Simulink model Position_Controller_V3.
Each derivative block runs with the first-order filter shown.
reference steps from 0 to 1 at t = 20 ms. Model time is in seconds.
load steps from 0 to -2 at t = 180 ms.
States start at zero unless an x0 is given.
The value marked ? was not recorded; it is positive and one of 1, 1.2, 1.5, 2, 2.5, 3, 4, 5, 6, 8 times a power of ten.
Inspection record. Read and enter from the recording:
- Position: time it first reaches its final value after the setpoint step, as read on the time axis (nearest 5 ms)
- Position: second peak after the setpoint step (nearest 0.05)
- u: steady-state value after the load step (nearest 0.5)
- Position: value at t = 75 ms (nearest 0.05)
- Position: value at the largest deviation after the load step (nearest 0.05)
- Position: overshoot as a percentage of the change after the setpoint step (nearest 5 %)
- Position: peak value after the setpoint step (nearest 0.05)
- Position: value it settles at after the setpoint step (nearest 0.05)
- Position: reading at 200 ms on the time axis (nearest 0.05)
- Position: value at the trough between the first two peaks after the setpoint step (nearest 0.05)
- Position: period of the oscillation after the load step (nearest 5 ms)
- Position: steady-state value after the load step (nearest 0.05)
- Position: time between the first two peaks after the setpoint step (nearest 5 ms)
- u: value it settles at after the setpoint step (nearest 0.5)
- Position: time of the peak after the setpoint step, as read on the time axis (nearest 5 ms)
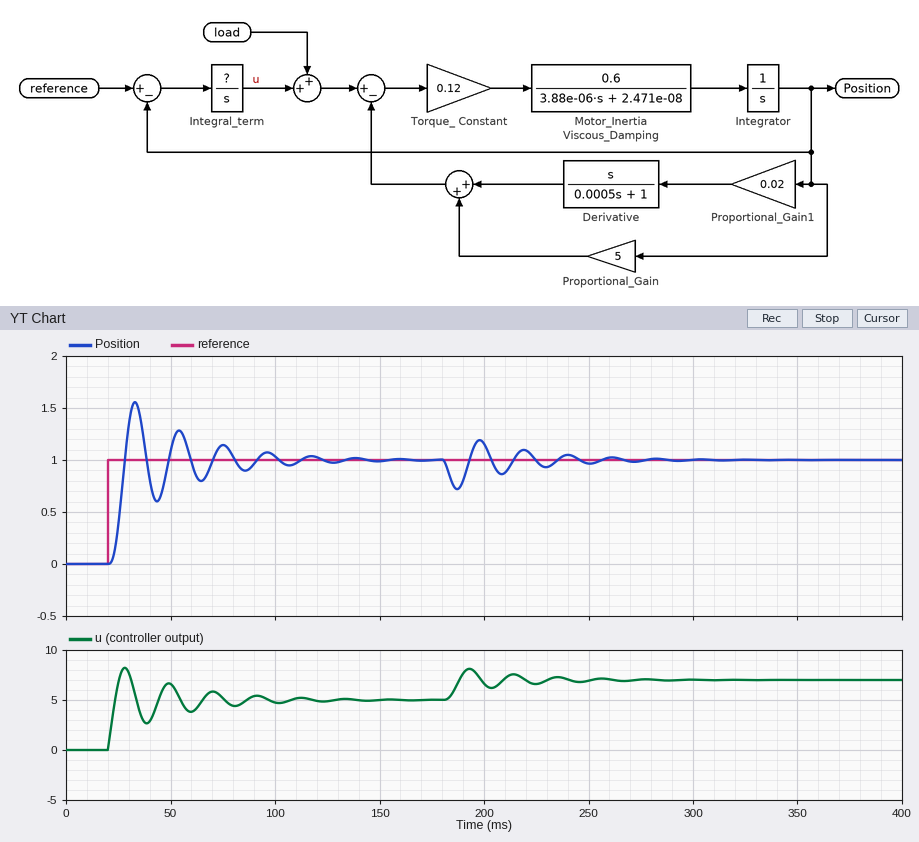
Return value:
30 ms
1.30
7.0
1.15
0.70
55 %
1.55
1.00
1.15
0.60
20 ms
1.00
20 ms
5.0
35 ms
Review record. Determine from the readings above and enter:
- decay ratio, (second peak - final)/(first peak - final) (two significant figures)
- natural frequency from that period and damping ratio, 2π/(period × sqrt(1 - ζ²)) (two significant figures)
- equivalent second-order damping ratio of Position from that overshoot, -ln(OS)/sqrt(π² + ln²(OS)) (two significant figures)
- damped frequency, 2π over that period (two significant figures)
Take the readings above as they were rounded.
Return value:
0.55
0.32 rad/ms
0.19
0.31 rad/ms
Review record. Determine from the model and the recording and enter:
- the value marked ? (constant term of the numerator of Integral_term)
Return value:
1500
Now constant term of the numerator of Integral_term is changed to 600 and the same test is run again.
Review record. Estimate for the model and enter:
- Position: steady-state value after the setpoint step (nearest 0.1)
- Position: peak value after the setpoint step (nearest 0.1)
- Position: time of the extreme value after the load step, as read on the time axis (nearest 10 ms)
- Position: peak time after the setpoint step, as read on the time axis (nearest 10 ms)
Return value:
1.0
1.1
190 ms
40 ms
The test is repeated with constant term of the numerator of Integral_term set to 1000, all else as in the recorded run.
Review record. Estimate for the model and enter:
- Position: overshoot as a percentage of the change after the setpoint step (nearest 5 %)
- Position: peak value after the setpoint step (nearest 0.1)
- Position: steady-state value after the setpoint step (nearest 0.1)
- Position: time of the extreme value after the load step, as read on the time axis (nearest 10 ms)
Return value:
30 %
1.3
1.0
190 ms
